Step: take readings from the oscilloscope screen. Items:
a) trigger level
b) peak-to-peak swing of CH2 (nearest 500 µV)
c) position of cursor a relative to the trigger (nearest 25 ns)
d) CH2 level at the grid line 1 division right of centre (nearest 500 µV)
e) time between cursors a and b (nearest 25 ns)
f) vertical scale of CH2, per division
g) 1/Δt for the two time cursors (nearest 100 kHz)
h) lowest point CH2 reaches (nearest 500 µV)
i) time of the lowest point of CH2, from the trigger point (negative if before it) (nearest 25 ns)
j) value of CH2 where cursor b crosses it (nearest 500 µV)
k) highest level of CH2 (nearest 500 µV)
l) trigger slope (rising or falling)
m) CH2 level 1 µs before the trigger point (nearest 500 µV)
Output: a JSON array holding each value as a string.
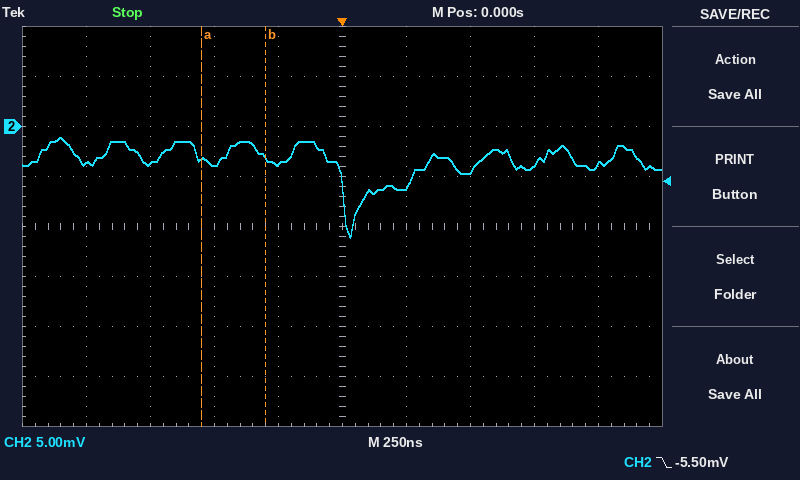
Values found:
["-5.50 mV", "10.0 mV", "-550 ns", "-6.0 mV", "250 ns", "5 mV", "4.0 MHz", "-11.0 mV", "+25 ns", "-3.0 mV", "-1.0 mV", "falling", "-3.5 mV"]
